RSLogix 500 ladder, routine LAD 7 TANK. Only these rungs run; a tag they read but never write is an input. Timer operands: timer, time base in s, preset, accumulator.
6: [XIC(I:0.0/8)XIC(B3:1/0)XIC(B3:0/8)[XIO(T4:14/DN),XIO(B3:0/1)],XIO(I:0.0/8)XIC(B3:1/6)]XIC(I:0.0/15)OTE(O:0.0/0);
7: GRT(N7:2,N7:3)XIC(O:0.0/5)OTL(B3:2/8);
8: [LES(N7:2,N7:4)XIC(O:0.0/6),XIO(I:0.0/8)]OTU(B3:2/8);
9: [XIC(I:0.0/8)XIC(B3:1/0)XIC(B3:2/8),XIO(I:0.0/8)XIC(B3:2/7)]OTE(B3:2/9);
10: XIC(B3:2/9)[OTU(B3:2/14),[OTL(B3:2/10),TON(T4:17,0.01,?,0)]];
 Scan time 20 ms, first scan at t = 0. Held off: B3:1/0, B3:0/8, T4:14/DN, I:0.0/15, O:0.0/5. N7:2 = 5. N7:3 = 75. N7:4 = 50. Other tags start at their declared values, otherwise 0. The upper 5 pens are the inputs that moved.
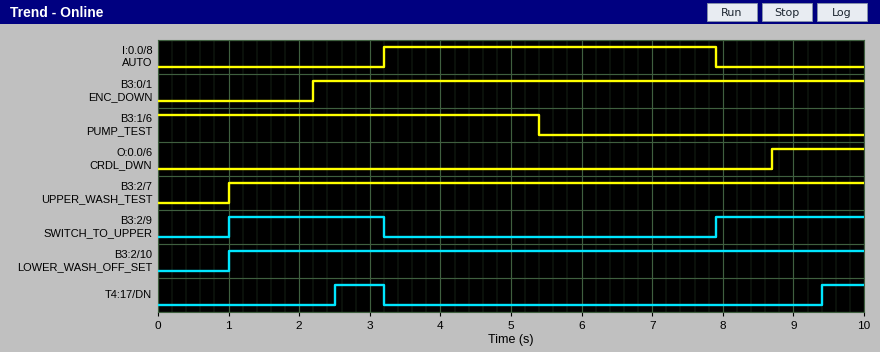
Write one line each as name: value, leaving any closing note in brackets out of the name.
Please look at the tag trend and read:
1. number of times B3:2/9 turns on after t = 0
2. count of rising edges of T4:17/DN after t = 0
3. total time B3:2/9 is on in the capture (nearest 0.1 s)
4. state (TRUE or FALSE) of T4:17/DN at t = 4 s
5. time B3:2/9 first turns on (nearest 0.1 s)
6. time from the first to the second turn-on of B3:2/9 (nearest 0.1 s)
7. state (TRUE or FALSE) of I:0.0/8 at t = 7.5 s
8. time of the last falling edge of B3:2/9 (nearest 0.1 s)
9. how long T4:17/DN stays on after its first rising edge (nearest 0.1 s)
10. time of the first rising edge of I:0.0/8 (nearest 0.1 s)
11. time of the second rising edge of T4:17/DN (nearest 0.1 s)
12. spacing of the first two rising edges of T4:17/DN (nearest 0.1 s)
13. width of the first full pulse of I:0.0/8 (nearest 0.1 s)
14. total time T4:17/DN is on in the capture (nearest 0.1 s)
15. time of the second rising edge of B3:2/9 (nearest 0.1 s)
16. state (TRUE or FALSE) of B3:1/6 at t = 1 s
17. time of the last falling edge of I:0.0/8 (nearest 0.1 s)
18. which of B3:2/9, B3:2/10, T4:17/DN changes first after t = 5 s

number of times B3:2/9 turns on after t = 0: 2
count of rising edges of T4:17/DN after t = 0: 2
total time B3:2/9 is on in the capture: 4.3 s
state (TRUE or FALSE) of T4:17/DN at t = 4 s: FALSE
time B3:2/9 first turns on: 1.0 s
time from the first to the second turn-on of B3:2/9: 6.9 s
state (TRUE or FALSE) of I:0.0/8 at t = 7.5 s: TRUE
time of the last falling edge of B3:2/9: 3.2 s
how long T4:17/DN stays on after its first rising edge: 0.7 s
time of the first rising edge of I:0.0/8: 3.2 s
time of the second rising edge of T4:17/DN: 9.4 s
spacing of the first two rising edges of T4:17/DN: 6.9 s
width of the first full pulse of I:0.0/8: 4.7 s
total time T4:17/DN is on in the capture: 1.3 s
time of the second rising edge of B3:2/9: 7.9 s
state (TRUE or FALSE) of B3:1/6 at t = 1 s: TRUE
time of the last falling edge of I:0.0/8: 7.9 s
which of B3:2/9, B3:2/10, T4:17/DN changes first after t = 5 s: B3:2/9
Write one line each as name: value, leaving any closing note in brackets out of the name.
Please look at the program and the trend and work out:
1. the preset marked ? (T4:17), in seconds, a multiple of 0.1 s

the preset marked ? (T4:17), in seconds, a multiple of 0.1 s: 1.5 s
